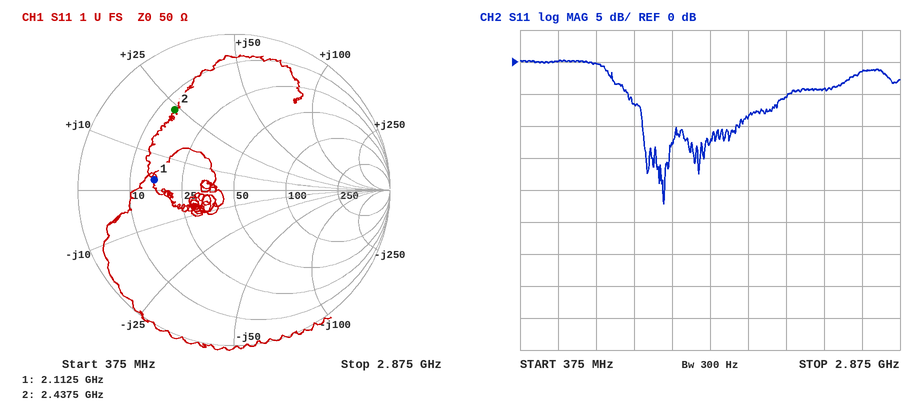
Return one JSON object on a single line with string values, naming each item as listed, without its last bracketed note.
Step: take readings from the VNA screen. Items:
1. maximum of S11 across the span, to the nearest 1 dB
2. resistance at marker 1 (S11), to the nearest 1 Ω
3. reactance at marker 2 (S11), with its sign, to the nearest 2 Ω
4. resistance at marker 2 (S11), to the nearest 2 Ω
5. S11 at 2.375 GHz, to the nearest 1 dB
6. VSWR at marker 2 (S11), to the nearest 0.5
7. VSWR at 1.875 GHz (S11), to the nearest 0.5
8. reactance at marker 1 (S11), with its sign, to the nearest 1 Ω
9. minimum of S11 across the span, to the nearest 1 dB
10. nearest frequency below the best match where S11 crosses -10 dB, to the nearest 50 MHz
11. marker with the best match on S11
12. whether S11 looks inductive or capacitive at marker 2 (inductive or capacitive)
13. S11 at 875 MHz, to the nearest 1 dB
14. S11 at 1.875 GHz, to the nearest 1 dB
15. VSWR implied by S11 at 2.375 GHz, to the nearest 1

{"maximum of S11 across the span, to the nearest 1 dB": "0 dB", "resistance at marker 1 (S11), to the nearest 1 Ω": "16 Ω", "reactance at marker 2 (S11), with its sign, to the nearest 2 Ω": "+24 Ω", "resistance at marker 2 (S11), to the nearest 2 Ω": "14 Ω", "S11 at 2.375 GHz, to the nearest 1 dB": "-4 dB", "VSWR at marker 2 (S11), to the nearest 0.5": "4.5", "VSWR at 1.875 GHz (S11), to the nearest 0.5": "2.0", "reactance at marker 1 (S11), with its sign, to the nearest 1 Ω": "+3 Ω", "minimum of S11 across the span, to the nearest 1 dB": "-22 dB", "nearest frequency below the best match where S11 crosses -10 dB, to the nearest 50 MHz": "1.20 GHz", "marker with the best match on S11": "marker 1", "whether S11 looks inductive or capacitive at marker 2": "inductive", "S11 at 875 MHz, to the nearest 1 dB": "0 dB", "S11 at 1.875 GHz, to the nearest 1 dB": "-9 dB", "VSWR implied by S11 at 2.375 GHz, to the nearest 1": "4"}
